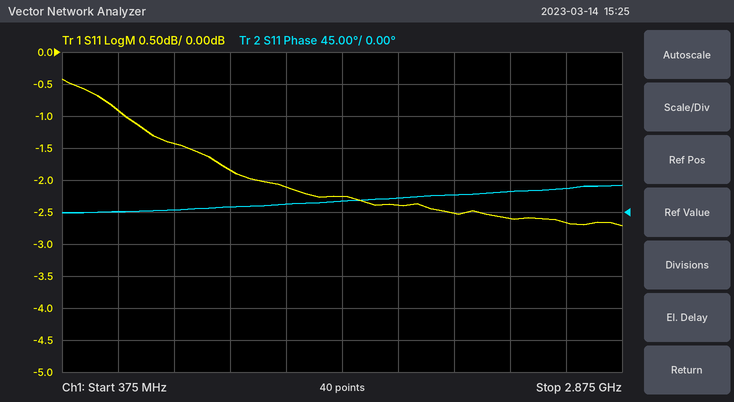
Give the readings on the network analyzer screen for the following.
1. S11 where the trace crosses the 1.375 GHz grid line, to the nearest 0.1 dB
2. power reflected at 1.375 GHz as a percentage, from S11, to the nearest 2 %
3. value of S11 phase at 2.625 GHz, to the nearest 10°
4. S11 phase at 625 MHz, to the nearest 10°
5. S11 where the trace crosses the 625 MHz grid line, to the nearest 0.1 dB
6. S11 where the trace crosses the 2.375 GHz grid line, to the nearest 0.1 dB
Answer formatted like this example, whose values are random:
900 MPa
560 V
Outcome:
-2.1 dB
62 %
30°
0°
-0.9 dB
-2.6 dB
